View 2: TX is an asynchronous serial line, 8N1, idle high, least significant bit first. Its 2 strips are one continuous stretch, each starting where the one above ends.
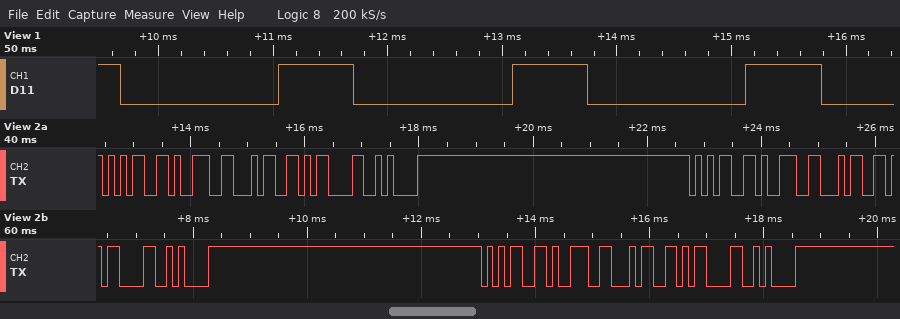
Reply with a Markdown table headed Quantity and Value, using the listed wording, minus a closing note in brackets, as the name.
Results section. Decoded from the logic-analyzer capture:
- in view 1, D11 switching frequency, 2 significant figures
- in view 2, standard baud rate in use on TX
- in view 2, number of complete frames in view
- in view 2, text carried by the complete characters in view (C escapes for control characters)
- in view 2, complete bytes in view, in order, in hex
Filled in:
| Quantity | Value |
|---|---|
| in view 1, D11 switching frequency, 2 significant figures | 490 Hz |
| in view 2, standard baud rate in use on TX | 9600 baud |
| in view 2, number of complete frames in view | 15 |
| in view 2, text carried by the complete characters in view | "594\r\n594\r\n594\r\n" |
| in view 2, complete bytes in view, in order, in hex | 35 39 34 0D 0A 35 39 34 0D 0A 35 39 34 0D 0A |
